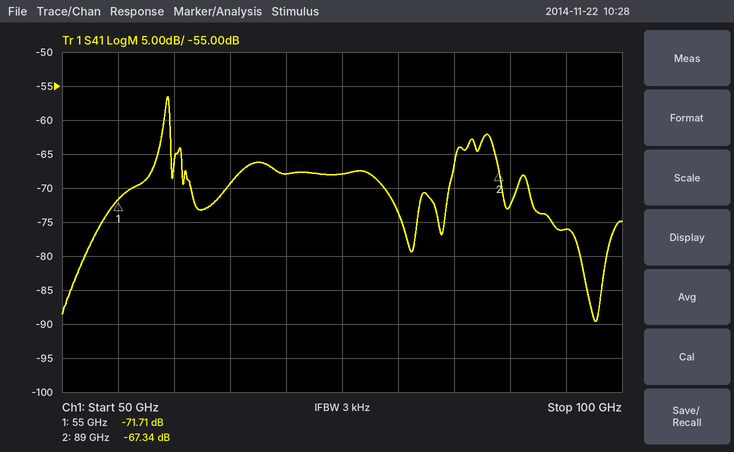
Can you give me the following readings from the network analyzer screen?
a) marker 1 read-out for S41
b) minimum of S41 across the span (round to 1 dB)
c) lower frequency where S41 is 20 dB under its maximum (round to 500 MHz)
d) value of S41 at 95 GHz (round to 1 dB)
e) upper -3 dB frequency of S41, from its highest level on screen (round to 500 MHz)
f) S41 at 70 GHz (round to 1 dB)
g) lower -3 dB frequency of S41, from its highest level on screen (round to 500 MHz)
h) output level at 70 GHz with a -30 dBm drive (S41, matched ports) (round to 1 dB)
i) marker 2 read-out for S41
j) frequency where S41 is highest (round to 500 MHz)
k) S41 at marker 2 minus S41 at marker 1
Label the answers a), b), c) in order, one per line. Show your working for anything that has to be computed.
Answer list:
a) -71.71 dB
b) -90 dB
c) 53.0 GHz
d) -76 dB
e) 59.5 GHz
f) -68 dB
g) 59.0 GHz
h) -30 dBm + (-68 dB) = -98 dBm
i) -67.34 dB
j) 59.5 GHz
k) -67.34 − (-71.71) = 4.37 dB
